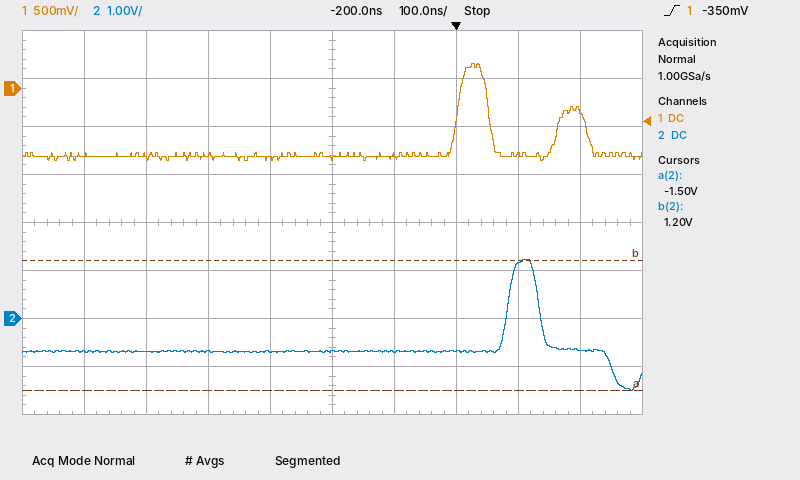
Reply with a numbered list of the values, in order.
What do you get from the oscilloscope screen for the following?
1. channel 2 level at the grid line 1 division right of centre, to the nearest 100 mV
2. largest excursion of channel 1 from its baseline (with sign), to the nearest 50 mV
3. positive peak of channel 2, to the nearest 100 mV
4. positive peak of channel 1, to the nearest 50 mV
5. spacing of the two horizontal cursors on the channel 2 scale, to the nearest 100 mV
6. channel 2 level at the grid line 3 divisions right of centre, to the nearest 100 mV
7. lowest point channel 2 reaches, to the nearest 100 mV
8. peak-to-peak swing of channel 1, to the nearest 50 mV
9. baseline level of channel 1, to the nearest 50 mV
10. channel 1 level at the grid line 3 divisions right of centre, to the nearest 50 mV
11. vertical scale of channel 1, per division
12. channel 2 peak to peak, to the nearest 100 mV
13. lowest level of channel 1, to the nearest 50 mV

1. -700 mV
2. +950 mV
3. 1.2 V
4. 250 mV
5. 2.7 V
6. 1.1 V
7. -1.5 V
8. 1.00 V
9. -700 mV
10. -700 mV
11. 500 mV
12. 2.7 V
13. -750 mV
